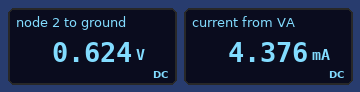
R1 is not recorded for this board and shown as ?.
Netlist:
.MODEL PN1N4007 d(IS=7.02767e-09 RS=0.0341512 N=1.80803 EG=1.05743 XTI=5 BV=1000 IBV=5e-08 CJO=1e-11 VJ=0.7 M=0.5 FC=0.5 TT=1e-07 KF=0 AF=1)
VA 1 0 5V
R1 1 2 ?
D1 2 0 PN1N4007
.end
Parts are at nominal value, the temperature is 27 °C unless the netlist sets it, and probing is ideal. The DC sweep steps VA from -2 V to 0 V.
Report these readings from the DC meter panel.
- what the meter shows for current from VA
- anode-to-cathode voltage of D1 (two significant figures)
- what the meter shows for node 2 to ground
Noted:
4.376 mA
620 mV
0.624 V
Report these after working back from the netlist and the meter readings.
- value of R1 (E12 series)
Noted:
1 kΩ
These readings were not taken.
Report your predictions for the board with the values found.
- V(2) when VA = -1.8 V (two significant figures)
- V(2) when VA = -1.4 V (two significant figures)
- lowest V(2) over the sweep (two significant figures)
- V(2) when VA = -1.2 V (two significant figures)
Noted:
-1.8 V
-1.4 V
-2.0 V
-1.2 V
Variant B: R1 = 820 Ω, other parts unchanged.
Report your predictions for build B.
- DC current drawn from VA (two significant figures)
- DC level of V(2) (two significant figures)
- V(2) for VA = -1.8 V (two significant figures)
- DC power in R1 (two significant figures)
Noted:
5.3 mA
630 mV
-1.8 V
23 mW
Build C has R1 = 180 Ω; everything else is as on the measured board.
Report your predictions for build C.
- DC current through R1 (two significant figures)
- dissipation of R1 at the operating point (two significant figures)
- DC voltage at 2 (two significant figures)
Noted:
24 mA
100 mW
700 mV
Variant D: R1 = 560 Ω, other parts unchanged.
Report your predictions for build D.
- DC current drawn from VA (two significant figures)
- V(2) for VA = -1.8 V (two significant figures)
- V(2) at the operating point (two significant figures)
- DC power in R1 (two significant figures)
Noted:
7.8 mA
-1.8 V
650 mV
34 mW
